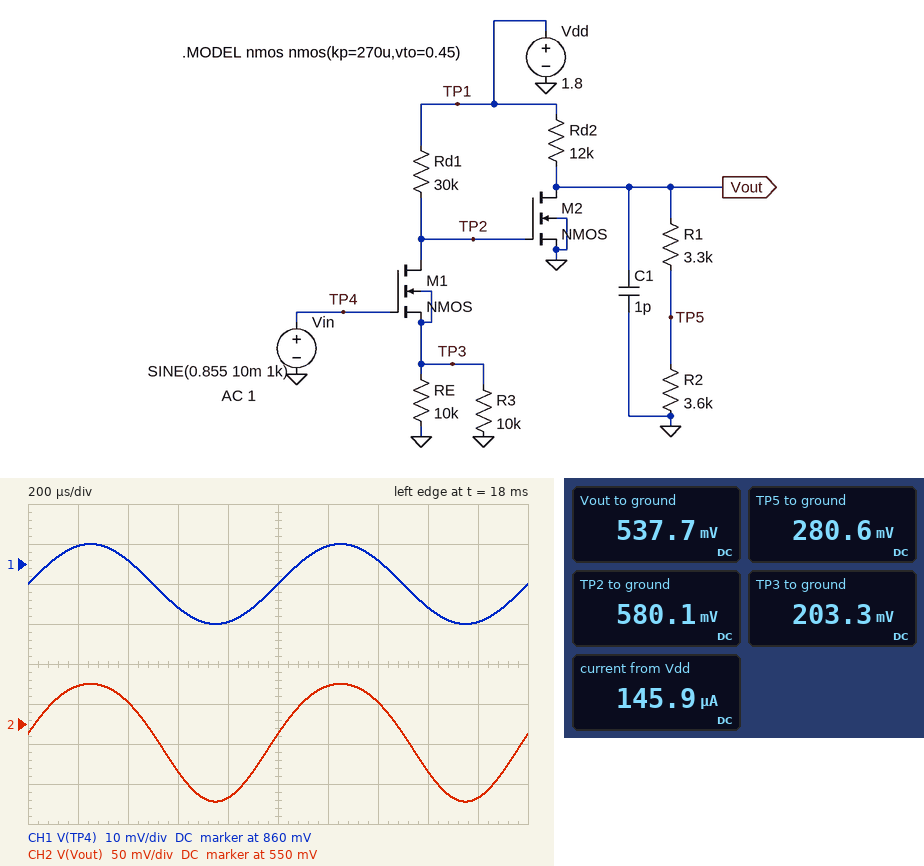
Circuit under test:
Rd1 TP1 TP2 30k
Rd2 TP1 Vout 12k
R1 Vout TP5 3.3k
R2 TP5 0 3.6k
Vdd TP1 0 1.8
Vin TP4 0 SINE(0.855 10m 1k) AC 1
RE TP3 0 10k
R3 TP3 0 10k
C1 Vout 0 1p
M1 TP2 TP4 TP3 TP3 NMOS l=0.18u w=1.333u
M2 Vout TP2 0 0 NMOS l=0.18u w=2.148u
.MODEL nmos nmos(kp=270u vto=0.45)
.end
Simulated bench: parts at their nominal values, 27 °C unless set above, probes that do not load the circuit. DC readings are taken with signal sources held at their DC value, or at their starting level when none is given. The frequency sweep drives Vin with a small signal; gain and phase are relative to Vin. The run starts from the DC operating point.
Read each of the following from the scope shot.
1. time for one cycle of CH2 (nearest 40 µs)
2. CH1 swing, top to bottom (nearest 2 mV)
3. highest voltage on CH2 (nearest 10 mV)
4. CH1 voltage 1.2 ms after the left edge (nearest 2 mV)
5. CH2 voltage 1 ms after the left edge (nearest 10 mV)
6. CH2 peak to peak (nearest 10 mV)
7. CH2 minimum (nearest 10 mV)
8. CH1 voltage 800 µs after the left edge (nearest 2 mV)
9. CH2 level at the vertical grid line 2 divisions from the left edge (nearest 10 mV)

1.00 ms
20 mV
600 mV
864 mV
540 mV
150 mV
450 mV
846 mV
580 mV
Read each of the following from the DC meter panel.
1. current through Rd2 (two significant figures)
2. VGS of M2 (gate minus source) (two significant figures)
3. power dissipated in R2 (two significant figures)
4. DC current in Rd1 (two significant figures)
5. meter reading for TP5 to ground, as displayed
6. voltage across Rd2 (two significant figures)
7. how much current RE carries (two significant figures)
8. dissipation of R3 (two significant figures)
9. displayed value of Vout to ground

110 µA
580 mV
22 µW
41 µA
280.6 mV
1.3 V
20 µA
4.1 µW
537.7 mV
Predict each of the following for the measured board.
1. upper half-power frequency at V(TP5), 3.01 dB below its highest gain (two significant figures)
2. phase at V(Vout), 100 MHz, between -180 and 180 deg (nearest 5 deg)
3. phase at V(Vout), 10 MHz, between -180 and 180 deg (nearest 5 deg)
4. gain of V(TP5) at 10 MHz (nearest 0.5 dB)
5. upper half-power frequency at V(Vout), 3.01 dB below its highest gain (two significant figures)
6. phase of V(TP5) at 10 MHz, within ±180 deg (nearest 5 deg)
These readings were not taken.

36 MHz
-70 deg
-15 deg
11.5 dB
36 MHz
-15 deg
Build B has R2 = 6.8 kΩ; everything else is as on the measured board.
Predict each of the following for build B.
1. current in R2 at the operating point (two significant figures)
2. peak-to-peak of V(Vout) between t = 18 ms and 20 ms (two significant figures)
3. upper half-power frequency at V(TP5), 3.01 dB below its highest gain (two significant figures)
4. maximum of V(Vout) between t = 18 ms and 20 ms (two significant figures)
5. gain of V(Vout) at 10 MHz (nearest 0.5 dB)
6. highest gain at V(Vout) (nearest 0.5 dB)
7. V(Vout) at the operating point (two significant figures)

67 µA
180 mV
29 MHz
750 mV
19.0 dB
19.5 dB
670 mV
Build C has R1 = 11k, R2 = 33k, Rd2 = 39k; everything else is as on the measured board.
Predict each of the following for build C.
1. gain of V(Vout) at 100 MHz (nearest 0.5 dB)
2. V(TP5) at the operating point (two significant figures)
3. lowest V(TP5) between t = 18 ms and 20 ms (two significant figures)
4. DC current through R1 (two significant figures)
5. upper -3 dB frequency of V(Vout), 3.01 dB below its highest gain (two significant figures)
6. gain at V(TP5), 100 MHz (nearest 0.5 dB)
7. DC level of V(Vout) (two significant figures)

8.5 dB
290 mV
83 mV
8.9 µA
7.7 MHz
6.0 dB
390 mV
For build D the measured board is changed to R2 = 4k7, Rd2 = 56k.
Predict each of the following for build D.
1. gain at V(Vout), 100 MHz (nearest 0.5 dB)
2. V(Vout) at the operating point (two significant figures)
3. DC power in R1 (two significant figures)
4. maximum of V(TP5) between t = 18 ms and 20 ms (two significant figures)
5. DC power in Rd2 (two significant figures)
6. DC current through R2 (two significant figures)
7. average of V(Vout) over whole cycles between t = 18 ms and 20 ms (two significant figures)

2.5 dB
72 mV
270 nW
79 mV
53 µW
9.0 µA
83 mV
